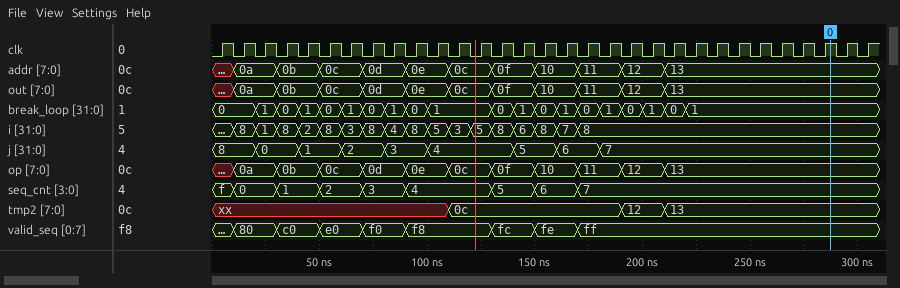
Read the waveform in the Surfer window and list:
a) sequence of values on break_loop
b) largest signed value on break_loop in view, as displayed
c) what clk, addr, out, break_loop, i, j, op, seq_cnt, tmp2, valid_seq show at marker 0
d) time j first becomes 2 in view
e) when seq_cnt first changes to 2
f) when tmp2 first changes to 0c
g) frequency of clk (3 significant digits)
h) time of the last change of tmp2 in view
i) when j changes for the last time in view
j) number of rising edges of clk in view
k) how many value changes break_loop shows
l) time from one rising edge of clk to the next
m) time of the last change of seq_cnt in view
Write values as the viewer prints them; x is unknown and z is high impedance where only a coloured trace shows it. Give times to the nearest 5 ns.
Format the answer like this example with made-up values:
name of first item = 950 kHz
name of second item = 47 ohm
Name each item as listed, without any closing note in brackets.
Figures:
sequence of values on break_loop = 0, 1, 0, 1, 0, 1, 0, 1, 0, 1, 0, 1, 0, 1, 0, 1, 0, 1, 0, 1
largest signed value on break_loop in view, as displayed = 1
what clk, addr, out, break_loop, i, j, op, seq_cnt, tmp2, valid_seq show at marker 0 = clk=1, addr=13, out=13, break_loop=1, i=8, j=7, op=13, seq_cnt=7, tmp2=13, valid_seq=ff
time j first becomes 2 in view = 60 ns
when seq_cnt first changes to 2 = 50 ns
when tmp2 first changes to 0c = 110 ns
frequency of clk = 100 MHz
time of the last change of tmp2 in view = 210 ns
when j changes for the last time in view = 180 ns
number of rising edges of clk in view = 31
how many value changes break_loop shows = 19
time from one rising edge of clk to the next = 10 ns
time of the last change of seq_cnt in view = 170 ns
